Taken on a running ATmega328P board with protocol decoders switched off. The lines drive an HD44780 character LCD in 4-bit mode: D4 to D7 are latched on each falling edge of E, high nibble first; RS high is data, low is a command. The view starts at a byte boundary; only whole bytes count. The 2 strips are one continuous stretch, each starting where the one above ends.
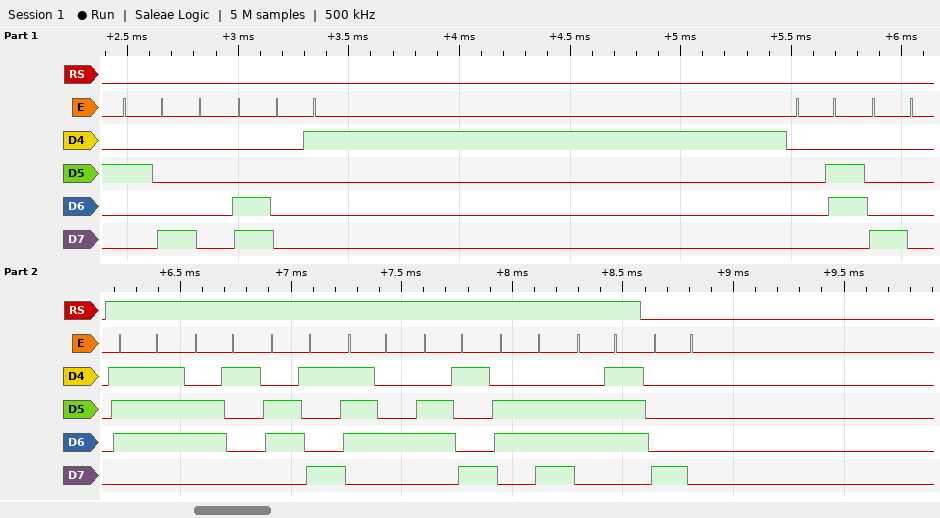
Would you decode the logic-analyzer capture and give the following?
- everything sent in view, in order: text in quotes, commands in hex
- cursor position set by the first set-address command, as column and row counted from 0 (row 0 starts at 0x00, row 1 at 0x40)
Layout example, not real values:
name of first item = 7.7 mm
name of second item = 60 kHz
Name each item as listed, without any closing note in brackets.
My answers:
everything sent in view, in order: text in quotes, commands in hex = 0x28 0x0C 0x01 0x06 0x80 "waiting" 0x80
cursor position set by the first set-address command, as column and row counted from 0 = column 0, row 0
